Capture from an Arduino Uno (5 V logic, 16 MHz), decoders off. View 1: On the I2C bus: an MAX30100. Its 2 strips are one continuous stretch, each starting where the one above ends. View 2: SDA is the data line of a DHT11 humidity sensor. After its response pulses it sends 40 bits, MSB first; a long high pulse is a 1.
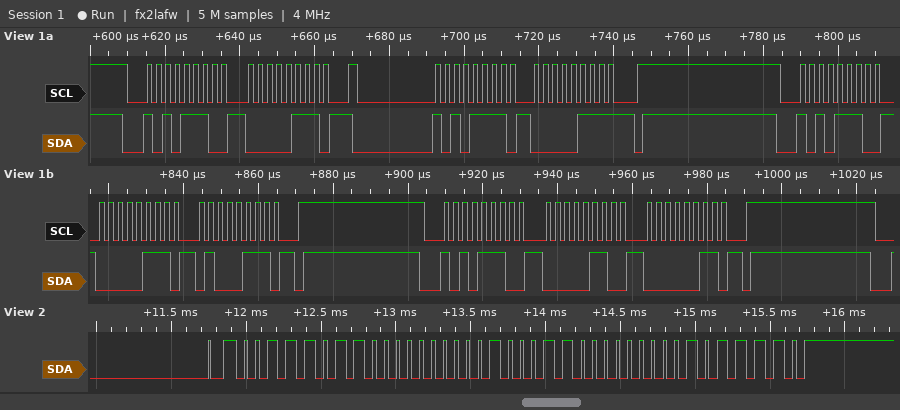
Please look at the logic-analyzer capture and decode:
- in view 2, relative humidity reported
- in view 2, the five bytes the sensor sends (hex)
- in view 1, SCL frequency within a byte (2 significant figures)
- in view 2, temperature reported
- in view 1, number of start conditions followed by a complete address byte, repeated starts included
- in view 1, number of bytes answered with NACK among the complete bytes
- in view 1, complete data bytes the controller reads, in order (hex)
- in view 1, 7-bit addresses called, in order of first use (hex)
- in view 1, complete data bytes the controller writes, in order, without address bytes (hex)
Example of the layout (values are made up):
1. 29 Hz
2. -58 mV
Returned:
1. 59 %
2. 3B 00 23 00 5E
3. 400 kHz
4. 35.0 °C
5. 4
6. 1
7. 07
8. 0x57
9. 07 07 47 06 03
